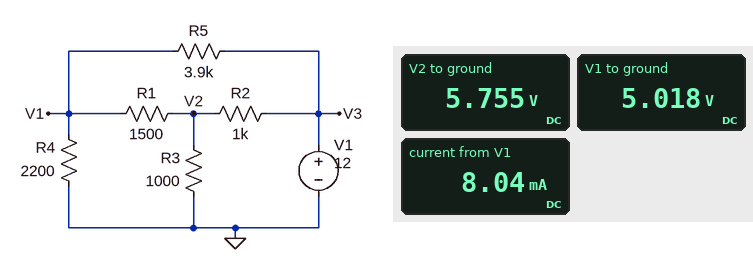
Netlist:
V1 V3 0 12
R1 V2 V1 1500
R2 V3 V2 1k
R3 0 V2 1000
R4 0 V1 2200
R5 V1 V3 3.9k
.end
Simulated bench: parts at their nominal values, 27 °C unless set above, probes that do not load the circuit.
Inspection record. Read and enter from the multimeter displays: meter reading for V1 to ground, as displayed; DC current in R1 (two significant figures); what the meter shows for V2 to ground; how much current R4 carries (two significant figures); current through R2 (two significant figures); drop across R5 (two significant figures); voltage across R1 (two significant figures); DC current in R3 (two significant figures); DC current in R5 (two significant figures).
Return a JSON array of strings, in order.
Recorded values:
["5.018 V", "490 µA", "5.755 V", "2.3 mA", "6.2 mA", "7.0 V", "740 mV", "5.8 mA", "1.8 mA"]
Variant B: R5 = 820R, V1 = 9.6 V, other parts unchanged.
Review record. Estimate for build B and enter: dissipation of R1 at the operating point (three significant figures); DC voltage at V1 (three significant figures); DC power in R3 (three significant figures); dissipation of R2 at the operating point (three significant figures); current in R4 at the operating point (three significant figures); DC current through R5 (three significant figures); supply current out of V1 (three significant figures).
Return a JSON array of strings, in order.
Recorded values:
["1.07 mW", "6.49 V", "27.3 mW", "19.2 mW", "2.95 mA", "3.79 mA", "8.17 mA"]
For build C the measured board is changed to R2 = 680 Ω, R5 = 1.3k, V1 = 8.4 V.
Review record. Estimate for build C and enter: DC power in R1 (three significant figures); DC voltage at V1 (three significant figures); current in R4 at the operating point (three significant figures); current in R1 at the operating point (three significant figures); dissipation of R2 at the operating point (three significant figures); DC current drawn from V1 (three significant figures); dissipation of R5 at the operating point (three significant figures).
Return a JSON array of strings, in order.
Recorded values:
["15.9 µW", "5.20 V", "2.36 mA", "103 µA", "16.6 mW", "7.40 mA", "7.90 mW"]
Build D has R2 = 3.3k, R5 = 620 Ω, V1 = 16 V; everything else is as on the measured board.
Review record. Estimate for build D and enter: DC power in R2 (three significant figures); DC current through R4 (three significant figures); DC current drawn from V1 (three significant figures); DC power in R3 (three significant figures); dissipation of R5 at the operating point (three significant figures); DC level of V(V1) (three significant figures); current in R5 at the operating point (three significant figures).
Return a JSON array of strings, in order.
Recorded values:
["29.3 mW", "4.97 mA", "11.1 mA", "38.0 mW", "41.3 mW", "10.9 V", "8.16 mA"]
